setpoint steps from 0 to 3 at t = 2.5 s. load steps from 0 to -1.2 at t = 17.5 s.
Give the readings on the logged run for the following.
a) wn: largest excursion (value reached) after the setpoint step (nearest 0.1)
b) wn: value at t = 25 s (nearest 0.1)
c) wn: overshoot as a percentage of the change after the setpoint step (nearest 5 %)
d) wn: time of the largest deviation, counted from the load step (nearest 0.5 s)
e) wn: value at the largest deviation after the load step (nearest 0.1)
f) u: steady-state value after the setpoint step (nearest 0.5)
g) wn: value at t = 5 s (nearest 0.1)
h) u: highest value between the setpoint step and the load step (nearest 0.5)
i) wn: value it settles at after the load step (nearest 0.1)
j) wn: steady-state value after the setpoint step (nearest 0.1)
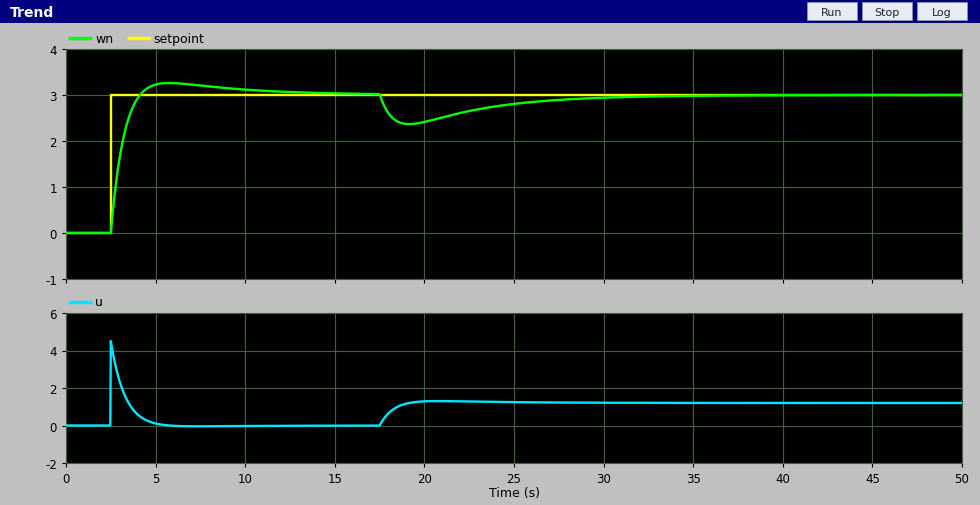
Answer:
3.3
2.8
10 %
1.5 s
2.4
0.0
3.2
4.5
3.0
3.0
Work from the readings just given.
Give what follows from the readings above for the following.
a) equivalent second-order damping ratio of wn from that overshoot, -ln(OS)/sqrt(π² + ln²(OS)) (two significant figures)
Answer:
0.59
